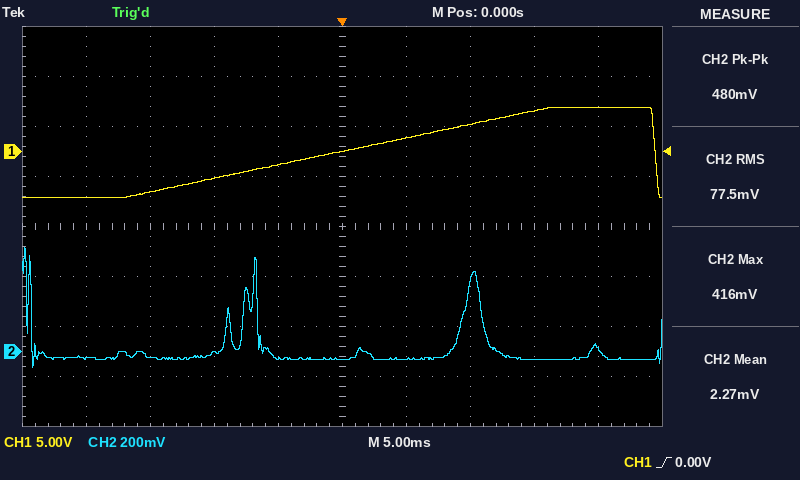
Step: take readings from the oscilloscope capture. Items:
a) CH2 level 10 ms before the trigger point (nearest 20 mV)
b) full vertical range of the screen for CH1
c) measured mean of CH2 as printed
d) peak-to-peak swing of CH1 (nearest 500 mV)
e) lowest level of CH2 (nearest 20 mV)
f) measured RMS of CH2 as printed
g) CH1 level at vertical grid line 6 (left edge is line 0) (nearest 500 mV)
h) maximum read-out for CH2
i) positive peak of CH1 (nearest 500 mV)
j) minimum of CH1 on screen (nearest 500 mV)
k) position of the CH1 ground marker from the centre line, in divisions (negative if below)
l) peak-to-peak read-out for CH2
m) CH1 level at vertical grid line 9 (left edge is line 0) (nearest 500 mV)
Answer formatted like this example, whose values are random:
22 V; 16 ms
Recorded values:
0 mV; 40 V; 2.27 mV; 9.0 V; -60 mV; 77.5 mV; 1.5 V; 416 mV; 4.5 V; -4.5 V; +1.5 div; 480 mV; 4.5 V
